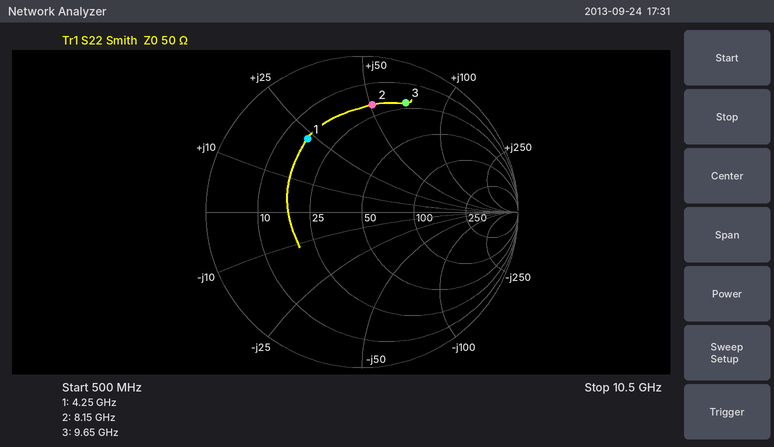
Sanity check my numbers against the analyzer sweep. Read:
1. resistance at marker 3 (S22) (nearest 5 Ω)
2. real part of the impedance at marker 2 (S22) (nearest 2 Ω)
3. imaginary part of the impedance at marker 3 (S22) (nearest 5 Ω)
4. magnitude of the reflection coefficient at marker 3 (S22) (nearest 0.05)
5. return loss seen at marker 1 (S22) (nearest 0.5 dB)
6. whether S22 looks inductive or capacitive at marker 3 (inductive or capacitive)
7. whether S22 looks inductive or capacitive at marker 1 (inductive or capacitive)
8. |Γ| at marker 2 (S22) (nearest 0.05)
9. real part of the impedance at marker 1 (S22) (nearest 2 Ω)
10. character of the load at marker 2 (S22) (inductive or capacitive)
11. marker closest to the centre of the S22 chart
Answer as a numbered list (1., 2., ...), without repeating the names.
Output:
1. 20 Ω
2. 20 Ω
3. +70 Ω
4. 0.75
5. 4.5 dB
6. inductive
7. inductive
8. 0.70
9. 16 Ω
10. inductive
11. marker 1
